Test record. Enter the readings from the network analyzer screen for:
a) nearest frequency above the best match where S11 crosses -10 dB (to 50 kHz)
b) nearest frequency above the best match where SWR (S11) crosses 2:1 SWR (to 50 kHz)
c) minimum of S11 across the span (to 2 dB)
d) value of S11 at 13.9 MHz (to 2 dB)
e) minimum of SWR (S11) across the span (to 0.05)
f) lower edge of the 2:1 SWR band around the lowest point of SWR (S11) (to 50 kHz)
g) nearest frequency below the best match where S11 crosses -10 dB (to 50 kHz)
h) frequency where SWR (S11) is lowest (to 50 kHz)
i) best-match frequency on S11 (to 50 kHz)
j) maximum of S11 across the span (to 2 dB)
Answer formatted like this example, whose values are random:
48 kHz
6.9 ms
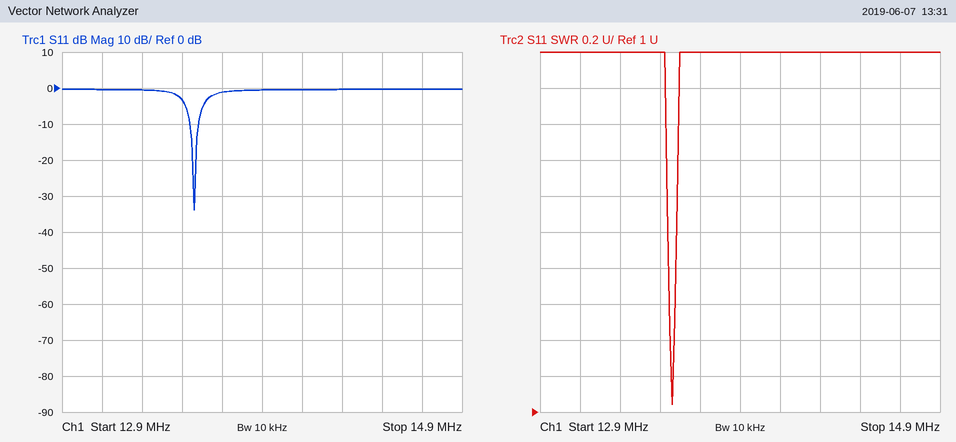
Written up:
13.60 MHz
13.60 MHz
-34 dB
0 dB
1.05
13.55 MHz
13.55 MHz
13.55 MHz
13.55 MHz
0 dB
